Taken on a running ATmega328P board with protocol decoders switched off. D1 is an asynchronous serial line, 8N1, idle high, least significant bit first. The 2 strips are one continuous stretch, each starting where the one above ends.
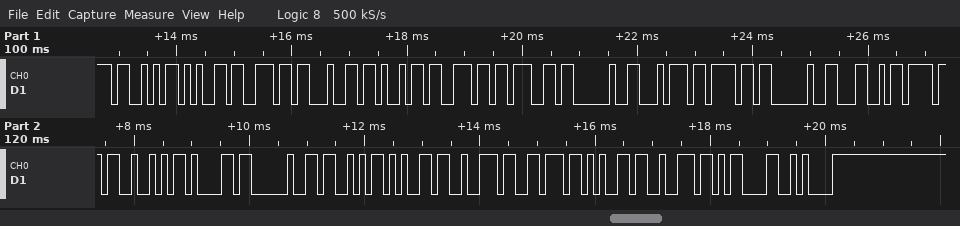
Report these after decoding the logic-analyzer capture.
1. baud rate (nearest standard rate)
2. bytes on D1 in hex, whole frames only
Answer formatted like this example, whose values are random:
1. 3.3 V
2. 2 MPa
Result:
1. 9600 baud
2. 0x53 0x65 0x6E 0x64 0x69 0x6E 0x67 0x20 0x74 0x6F 0x20 0x4C 0x6F 0x52 0x61 0x20 0x53 0x65 0x72 0x76 0x65 0x72 0x0D 0x0A
